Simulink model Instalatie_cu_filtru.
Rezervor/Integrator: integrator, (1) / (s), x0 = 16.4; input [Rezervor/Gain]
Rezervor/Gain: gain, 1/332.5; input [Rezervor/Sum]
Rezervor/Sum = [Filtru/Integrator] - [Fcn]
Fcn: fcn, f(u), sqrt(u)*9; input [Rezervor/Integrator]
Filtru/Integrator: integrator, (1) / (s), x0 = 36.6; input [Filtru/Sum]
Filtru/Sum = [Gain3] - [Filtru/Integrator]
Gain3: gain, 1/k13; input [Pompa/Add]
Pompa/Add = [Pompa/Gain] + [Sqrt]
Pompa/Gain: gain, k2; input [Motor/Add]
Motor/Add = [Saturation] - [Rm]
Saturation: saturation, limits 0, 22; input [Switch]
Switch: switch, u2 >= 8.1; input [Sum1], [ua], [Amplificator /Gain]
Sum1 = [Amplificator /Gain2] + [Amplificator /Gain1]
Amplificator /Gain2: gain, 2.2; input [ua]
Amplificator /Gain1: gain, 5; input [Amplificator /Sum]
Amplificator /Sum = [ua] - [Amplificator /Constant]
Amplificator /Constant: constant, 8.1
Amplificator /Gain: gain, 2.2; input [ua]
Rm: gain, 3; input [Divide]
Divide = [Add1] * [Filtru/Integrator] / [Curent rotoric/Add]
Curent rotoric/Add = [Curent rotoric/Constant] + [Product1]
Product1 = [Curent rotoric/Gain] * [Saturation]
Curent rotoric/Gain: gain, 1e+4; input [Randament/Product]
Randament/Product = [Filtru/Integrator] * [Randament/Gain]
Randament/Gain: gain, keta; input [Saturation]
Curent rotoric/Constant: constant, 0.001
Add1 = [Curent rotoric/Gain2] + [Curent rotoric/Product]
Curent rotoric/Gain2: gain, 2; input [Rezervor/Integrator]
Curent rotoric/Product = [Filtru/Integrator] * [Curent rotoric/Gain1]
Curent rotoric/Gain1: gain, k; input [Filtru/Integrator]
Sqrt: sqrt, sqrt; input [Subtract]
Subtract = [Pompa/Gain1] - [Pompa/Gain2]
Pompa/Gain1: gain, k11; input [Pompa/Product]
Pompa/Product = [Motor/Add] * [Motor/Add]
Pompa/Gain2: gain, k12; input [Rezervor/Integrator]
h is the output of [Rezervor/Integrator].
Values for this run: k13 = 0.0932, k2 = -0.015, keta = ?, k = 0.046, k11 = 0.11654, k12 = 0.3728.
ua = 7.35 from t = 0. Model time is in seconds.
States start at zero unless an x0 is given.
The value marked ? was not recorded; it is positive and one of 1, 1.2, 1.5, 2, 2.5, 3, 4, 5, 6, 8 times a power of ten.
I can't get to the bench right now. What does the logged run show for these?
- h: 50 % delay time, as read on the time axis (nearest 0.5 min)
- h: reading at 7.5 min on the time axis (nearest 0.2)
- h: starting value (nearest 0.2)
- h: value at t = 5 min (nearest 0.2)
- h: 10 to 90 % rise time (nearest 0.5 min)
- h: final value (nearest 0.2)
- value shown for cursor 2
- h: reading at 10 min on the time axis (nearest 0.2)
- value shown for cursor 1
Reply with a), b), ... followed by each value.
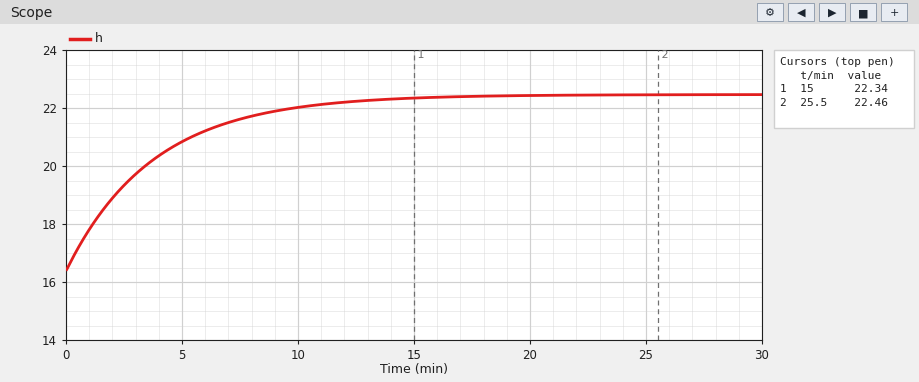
a) 2.5 min
b) 21.6
c) 16.4
d) 20.8
e) 8.5 min
f) 22.4
g) 22.46
h) 22.0
i) 22.34
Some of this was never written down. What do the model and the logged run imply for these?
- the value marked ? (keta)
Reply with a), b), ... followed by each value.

a) 0.00012
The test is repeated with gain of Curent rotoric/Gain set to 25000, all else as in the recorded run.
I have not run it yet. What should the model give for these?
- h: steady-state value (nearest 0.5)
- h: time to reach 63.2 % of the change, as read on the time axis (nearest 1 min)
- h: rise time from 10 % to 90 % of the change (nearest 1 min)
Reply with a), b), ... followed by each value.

a) 24.5
b) 4 min
c) 9 min
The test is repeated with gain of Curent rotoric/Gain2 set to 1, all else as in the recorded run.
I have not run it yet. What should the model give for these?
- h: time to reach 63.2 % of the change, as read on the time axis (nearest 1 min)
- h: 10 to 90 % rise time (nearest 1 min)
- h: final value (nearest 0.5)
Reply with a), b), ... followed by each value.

a) 4 min
b) 9 min
c) 23.0
